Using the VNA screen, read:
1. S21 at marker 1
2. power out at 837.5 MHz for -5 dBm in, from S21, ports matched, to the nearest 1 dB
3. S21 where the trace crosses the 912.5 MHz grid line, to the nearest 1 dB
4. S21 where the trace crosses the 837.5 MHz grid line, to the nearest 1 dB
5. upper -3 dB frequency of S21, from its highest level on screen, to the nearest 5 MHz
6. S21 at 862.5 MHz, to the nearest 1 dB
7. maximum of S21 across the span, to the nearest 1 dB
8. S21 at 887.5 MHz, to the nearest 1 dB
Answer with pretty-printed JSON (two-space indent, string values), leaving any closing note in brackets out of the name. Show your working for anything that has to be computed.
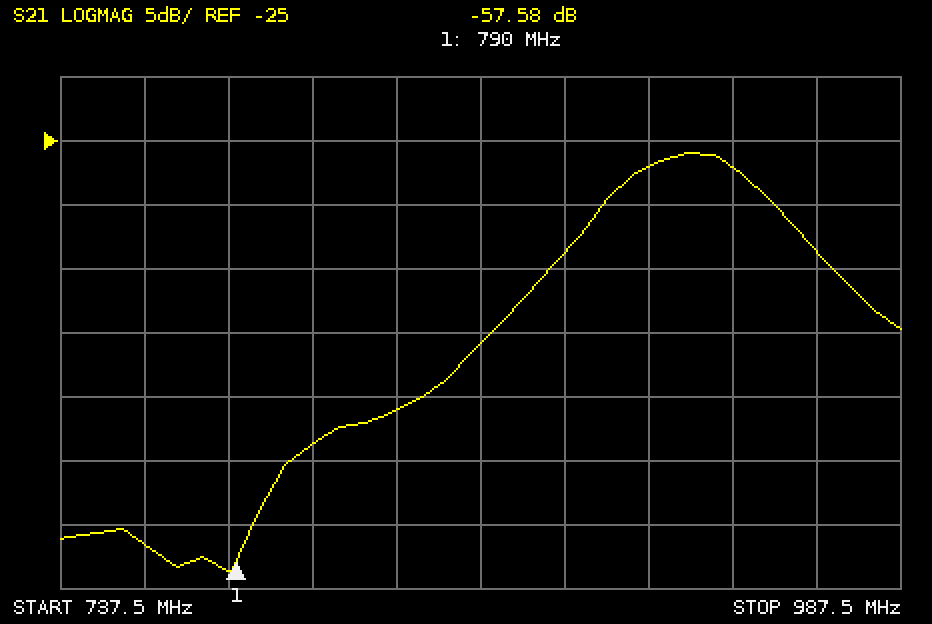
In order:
{
  "S21 at marker 1": "-57.58 dB",
  "power out at 837.5 MHz for -5 dBm in, from S21, ports matched, to the nearest 1 dB": "-5 dBm + (-46 dB) = -51 dBm",
  "S21 where the trace crosses the 912.5 MHz grid line, to the nearest 1 dB": "-27 dB",
  "S21 where the trace crosses the 837.5 MHz grid line, to the nearest 1 dB": "-46 dB",
  "upper -3 dB frequency of S21, from its highest level on screen, to the nearest 5 MHz": "945 MHz",
  "S21 at 862.5 MHz, to the nearest 1 dB": "-41 dB",
  "maximum of S21 across the span, to the nearest 1 dB": "-26 dB",
  "S21 at 887.5 MHz, to the nearest 1 dB": "-34 dB"
}
